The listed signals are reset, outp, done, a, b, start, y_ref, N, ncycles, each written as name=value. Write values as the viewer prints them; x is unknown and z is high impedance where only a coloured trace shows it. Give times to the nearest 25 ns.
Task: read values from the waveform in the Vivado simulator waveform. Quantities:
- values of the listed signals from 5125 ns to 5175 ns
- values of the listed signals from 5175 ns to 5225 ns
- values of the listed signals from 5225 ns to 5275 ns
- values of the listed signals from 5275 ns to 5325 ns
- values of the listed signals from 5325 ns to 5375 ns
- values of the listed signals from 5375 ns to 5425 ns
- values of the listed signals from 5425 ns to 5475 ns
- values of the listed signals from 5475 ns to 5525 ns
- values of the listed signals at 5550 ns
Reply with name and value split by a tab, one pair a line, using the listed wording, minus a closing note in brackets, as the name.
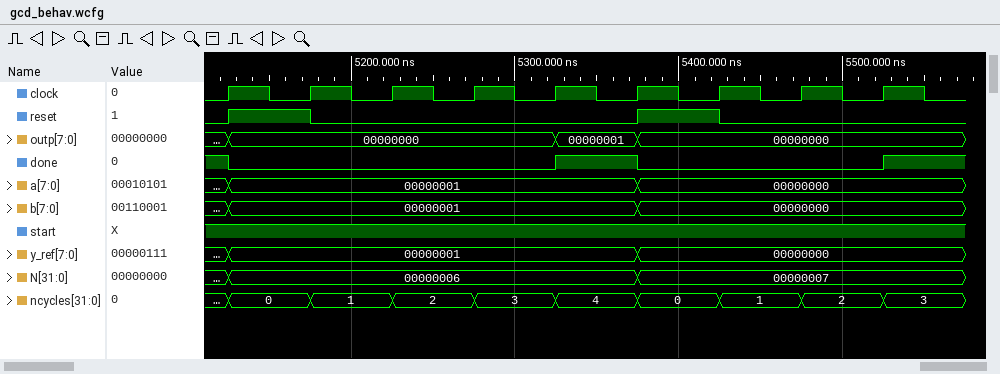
values of the listed signals from 5125 ns to 5175 ns	reset=1, outp=00000000, done=0, a=00000001, b=00000001, start=1, y_ref=00000001, N=00000006, ncycles=0
values of the listed signals from 5175 ns to 5225 ns	reset=0, outp=00000000, done=0, a=00000001, b=00000001, start=1, y_ref=00000001, N=00000006, ncycles=1
values of the listed signals from 5225 ns to 5275 ns	reset=0, outp=00000000, done=0, a=00000001, b=00000001, start=1, y_ref=00000001, N=00000006, ncycles=2
values of the listed signals from 5275 ns to 5325 ns	reset=0, outp=00000000, done=0, a=00000001, b=00000001, start=1, y_ref=00000001, N=00000006, ncycles=3
values of the listed signals from 5325 ns to 5375 ns	reset=0, outp=00000001, done=1, a=00000001, b=00000001, start=1, y_ref=00000001, N=00000006, ncycles=4
values of the listed signals from 5375 ns to 5425 ns	reset=1, outp=00000000, done=0, a=00000000, b=00000000, start=1, y_ref=00000000, N=00000007, ncycles=0
values of the listed signals from 5425 ns to 5475 ns	reset=0, outp=00000000, done=0, a=00000000, b=00000000, start=1, y_ref=00000000, N=00000007, ncycles=1
values of the listed signals from 5475 ns to 5525 ns	reset=0, outp=00000000, done=0, a=00000000, b=00000000, start=1, y_ref=00000000, N=00000007, ncycles=2
values of the listed signals at 5550 ns	reset=0, outp=00000000, done=1, a=00000000, b=00000000, start=1, y_ref=00000000, N=00000007, ncycles=3
